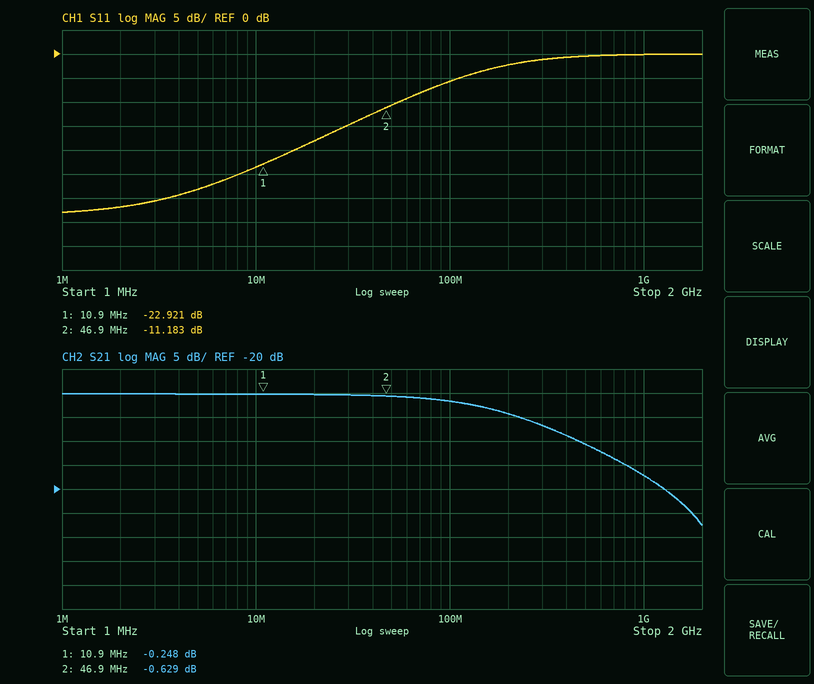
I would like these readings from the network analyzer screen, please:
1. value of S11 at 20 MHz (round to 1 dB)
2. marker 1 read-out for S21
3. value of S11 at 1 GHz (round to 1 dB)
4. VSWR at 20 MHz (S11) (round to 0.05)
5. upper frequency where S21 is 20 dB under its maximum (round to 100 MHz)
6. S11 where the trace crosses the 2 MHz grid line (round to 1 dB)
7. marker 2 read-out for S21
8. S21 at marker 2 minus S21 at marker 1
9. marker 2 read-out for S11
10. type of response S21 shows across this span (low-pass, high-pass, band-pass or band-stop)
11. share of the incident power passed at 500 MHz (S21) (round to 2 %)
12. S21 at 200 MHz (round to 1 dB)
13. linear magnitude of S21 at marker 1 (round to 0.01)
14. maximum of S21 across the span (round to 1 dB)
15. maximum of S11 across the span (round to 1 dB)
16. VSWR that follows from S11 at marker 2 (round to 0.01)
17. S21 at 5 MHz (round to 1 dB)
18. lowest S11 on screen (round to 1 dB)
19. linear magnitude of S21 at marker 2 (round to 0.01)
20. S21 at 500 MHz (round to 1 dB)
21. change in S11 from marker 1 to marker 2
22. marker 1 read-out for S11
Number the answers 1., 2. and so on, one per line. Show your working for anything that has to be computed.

1. -18 dB
2. -0.248 dB
3. 0 dB
4. |Γ| = 10^(-18/20) = 0.1259; VSWR = (1 + 0.1259)/(1 − 0.1259) ≈ 1.29, so 1.30 to the nearest 0.05
5. 1.3 GHz
6. -32 dB
7. -0.629 dB
8. -0.629 − (-0.248) = -0.381 dB
9. -11.183 dB
10. low-pass
11. 10^(-11/10) ≈ 8 %
12. -4 dB
13. 10^(-0.248/20) ≈ 0.97
14. 0 dB
15. 0 dB
16. (1 + 0.2760)/(1 − 0.2760) ≈ 1.76
17. 0 dB
18. -33 dB
19. 10^(-0.629/20) ≈ 0.93
20. -11 dB
21. -11.183 − (-22.921) = 11.738 dB
22. -22.921 dB
